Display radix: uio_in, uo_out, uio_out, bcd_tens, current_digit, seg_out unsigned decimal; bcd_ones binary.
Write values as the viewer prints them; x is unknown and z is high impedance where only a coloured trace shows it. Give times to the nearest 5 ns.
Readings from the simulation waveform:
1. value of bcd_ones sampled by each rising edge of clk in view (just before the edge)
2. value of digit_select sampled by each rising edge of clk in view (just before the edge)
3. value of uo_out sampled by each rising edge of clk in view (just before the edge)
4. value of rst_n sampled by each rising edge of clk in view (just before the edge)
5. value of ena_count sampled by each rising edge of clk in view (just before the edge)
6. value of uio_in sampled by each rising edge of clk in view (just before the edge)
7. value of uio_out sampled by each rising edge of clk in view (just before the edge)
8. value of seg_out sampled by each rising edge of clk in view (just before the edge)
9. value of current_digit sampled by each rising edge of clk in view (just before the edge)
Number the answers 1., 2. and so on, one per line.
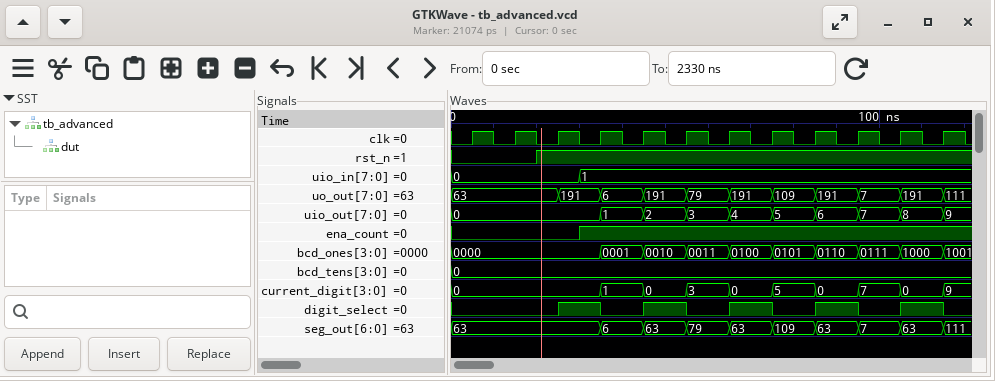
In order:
1. 0000, 0000, 0000, 0000, 0001, 0010, 0011, 0100, 0101, 0110, 0111, 1000
2. 0 0 0 1 0 1 0 1 0 1 0 1
3. 63, 63, 63, 191, 6, 191, 79, 191, 109, 191, 7, 191
4. 0 0 1 1 1 1 1 1 1 1 1 1
5. 0 0 0 1 1 1 1 1 1 1 1 1
6. 0, 0, 0, 1, 1, 1, 1, 1, 1, 1, 1, 1
7. 0, 0, 0, 0, 1, 2, 3, 4, 5, 6, 7, 8
8. 63, 63, 63, 63, 6, 63, 79, 63, 109, 63, 7, 63
9. 0, 0, 0, 0, 1, 0, 3, 0, 5, 0, 7, 0
